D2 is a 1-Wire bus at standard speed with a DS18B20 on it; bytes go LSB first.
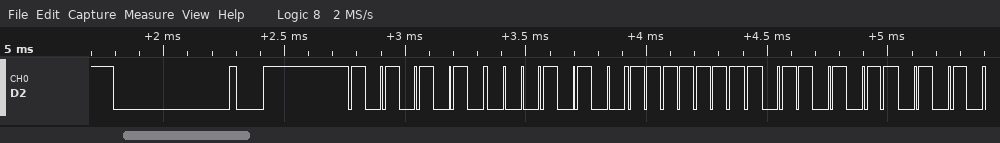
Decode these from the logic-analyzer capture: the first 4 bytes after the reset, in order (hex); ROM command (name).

55 28 FF D6
Match ROM
